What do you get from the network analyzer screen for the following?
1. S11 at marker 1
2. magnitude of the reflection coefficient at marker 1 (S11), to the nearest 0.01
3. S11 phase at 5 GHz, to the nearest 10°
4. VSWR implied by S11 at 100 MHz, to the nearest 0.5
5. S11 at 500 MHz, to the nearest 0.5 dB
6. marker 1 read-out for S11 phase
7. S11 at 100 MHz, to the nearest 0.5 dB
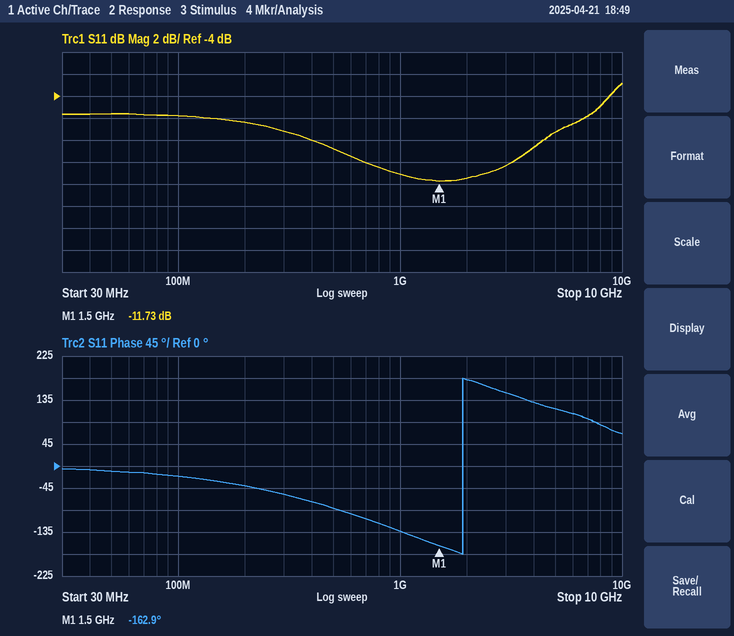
-11.73 dB
0.26
120°
3.0
-9.0 dB
-162.9°
-6.0 dB
